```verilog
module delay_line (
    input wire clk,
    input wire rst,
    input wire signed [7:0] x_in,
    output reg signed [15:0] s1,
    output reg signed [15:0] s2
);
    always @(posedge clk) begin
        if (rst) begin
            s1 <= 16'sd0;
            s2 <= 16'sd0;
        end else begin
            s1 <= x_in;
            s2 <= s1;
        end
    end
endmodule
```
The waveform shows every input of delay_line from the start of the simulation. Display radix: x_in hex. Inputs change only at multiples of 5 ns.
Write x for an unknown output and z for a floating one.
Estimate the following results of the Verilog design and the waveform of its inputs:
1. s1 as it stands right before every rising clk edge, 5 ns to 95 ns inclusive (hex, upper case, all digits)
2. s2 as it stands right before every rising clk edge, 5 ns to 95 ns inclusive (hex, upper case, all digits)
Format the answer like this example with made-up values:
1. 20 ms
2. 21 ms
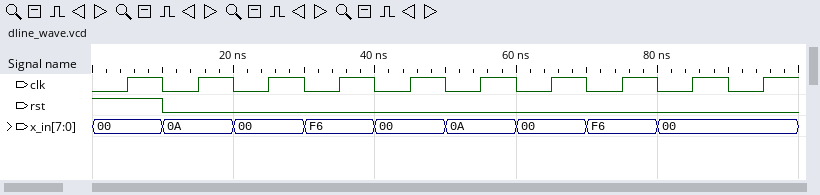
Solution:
1. x, 0000, 000A, 0000, FFF6, 0000, 000A, 0000, FFF6, 0000
2. x, 0000, 0000, 000A, 0000, FFF6, 0000, 000A, 0000, FFF6
